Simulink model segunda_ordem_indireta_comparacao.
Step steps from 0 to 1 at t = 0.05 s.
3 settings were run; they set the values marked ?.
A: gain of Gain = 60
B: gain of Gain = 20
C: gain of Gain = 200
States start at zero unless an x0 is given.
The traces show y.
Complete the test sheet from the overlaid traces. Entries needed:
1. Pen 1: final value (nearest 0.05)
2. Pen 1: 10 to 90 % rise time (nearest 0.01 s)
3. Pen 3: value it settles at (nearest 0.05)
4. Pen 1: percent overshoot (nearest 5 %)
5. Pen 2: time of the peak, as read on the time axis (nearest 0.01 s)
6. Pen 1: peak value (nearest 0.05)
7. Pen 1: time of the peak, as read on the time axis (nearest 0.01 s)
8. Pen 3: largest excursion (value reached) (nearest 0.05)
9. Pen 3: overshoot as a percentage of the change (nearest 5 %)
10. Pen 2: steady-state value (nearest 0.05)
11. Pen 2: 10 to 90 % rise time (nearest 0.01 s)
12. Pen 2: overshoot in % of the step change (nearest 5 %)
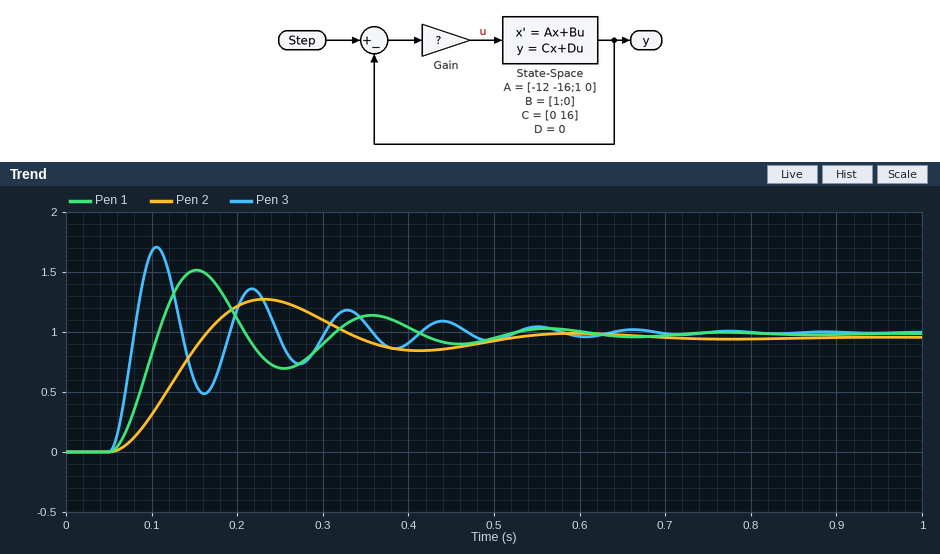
1.00
0.04 s
1.00
55 %
0.23 s
1.50
0.15 s
1.70
70 %
0.95
0.07 s
35 %
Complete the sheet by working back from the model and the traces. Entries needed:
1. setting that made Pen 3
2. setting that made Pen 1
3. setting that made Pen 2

C
A
B
